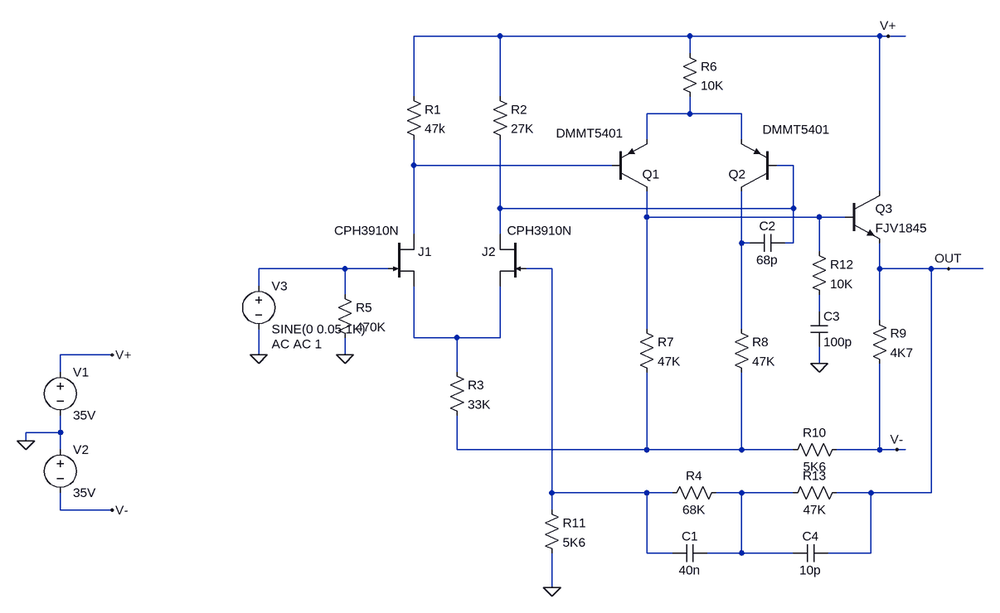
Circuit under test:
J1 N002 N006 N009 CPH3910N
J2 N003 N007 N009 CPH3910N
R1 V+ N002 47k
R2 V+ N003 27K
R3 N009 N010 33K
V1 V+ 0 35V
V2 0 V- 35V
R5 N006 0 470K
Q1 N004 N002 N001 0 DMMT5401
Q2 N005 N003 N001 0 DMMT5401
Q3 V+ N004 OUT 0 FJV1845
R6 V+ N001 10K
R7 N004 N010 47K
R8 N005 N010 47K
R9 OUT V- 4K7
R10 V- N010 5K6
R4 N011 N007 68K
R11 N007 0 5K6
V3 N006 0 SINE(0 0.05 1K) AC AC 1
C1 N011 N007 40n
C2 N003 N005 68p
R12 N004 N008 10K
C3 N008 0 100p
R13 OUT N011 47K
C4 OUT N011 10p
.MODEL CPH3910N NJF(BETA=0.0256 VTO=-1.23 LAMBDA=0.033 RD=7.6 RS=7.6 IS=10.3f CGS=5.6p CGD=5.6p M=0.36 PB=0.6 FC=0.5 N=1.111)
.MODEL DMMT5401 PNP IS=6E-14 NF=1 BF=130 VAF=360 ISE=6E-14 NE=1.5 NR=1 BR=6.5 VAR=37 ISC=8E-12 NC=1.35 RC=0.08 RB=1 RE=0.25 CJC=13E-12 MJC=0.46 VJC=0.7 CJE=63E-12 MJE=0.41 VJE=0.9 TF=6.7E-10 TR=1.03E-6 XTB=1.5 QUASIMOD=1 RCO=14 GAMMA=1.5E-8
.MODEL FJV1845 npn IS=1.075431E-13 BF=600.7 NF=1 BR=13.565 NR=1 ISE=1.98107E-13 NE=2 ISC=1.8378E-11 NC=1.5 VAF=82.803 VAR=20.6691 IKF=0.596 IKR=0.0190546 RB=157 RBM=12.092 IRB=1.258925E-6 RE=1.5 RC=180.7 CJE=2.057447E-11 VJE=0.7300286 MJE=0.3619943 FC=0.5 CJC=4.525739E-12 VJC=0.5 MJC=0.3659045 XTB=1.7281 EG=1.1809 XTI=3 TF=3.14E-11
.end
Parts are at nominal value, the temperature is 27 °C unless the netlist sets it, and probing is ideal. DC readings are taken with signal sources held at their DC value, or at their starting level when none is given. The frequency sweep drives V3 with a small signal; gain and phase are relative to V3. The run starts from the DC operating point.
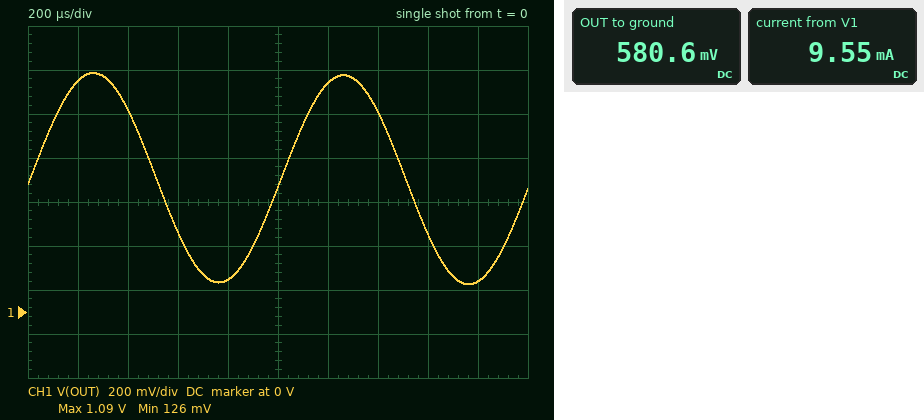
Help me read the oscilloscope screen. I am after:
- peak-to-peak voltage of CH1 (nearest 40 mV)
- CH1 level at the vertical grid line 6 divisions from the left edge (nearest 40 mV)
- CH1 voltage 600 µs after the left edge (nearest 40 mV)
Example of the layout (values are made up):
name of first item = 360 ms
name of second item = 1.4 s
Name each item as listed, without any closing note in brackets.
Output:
peak-to-peak voltage of CH1 = 960 mV
CH1 level at the vertical grid line 6 divisions from the left edge = 1.04 V
CH1 voltage 600 µs after the left edge = 360 mV
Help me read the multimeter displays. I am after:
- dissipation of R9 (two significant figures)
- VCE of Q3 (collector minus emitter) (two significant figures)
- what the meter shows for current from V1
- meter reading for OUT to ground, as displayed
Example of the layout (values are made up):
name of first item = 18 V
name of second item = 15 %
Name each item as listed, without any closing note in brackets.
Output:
dissipation of R9 = 270 mW
VCE of Q3 (collector minus emitter) = 34 V
what the meter shows for current from V1 = 9.55 mA
meter reading for OUT to ground, as displayed = 580.6 mV
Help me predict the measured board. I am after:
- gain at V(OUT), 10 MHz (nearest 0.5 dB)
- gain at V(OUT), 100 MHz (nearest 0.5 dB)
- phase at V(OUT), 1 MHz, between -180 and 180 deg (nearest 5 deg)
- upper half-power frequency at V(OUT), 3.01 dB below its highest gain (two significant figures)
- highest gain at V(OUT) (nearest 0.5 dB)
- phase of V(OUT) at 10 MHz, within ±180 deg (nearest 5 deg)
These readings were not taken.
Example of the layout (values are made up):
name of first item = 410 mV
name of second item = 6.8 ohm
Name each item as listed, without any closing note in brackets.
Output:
gain at V(OUT), 10 MHz = 1.5 dB
gain at V(OUT), 100 MHz = -10.5 dB
phase at V(OUT), 1 MHz, between -180 and 180 deg = -50 deg
upper half-power frequency at V(OUT), 3.01 dB below its highest gain = 74 Hz
highest gain at V(OUT) = 26.5 dB
phase of V(OUT) at 10 MHz, within ±180 deg = -25 deg
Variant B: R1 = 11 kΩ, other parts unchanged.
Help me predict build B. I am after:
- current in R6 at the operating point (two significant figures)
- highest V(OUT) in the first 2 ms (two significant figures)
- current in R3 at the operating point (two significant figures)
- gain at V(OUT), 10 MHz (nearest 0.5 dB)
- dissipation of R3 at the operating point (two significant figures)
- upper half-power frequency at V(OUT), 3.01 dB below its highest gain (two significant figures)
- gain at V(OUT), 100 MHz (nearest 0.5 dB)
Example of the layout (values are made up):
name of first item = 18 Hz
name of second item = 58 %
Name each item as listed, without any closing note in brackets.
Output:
current in R6 at the operating point = 600 µA
highest V(OUT) in the first 2 ms = -440 mV
current in R3 at the operating point = 850 µA
gain at V(OUT), 10 MHz = 1.0 dB
dissipation of R3 at the operating point = 24 mW
upper half-power frequency at V(OUT), 3.01 dB below its highest gain = 75 Hz
gain at V(OUT), 100 MHz = -1.5 dB
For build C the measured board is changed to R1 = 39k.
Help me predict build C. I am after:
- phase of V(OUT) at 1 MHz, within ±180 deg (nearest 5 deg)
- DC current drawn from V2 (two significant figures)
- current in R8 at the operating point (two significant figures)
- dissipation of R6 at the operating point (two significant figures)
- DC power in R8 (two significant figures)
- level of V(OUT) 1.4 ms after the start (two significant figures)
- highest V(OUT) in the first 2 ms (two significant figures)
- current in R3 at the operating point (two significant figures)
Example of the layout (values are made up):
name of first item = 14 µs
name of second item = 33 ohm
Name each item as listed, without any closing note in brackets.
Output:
phase of V(OUT) at 1 MHz, within ±180 deg = -50 deg
DC current drawn from V2 = 9.4 mA
current in R8 at the operating point = 600 µA
dissipation of R6 at the operating point = 13 mW
DC power in R8 = 17 mW
level of V(OUT) 1.4 ms after the start = 720 mV
highest V(OUT) in the first 2 ms = 890 mV
current in R3 at the operating point = 770 µA
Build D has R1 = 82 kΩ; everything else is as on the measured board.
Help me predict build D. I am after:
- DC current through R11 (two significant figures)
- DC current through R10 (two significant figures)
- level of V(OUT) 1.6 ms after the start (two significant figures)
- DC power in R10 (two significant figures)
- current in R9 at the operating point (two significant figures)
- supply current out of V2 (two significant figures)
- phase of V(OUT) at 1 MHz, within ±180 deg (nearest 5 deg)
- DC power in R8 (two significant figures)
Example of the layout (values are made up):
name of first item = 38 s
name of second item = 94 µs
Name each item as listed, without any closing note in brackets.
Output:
DC current through R11 = 9.2 µA
DC current through R10 = 2.1 mA
level of V(OUT) 1.6 ms after the start = 880 mV
DC power in R10 = 25 mW
current in R9 at the operating point = 7.7 mA
supply current out of V2 = 9.8 mA
phase of V(OUT) at 1 MHz, within ±180 deg = -50 deg
DC power in R8 = 35 mW
